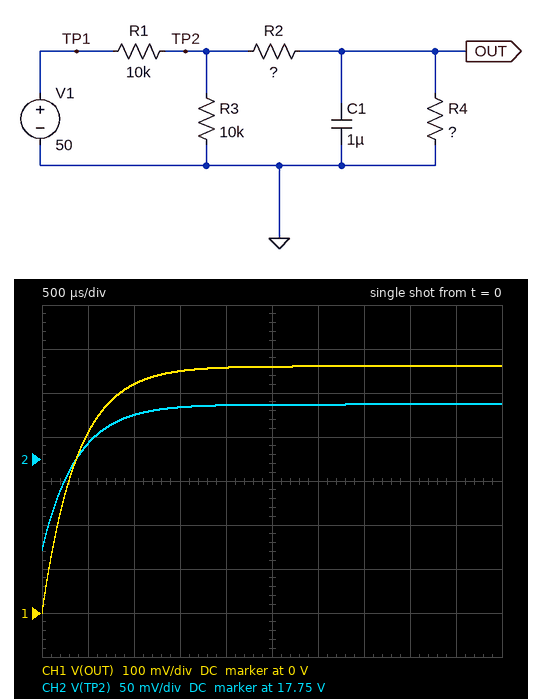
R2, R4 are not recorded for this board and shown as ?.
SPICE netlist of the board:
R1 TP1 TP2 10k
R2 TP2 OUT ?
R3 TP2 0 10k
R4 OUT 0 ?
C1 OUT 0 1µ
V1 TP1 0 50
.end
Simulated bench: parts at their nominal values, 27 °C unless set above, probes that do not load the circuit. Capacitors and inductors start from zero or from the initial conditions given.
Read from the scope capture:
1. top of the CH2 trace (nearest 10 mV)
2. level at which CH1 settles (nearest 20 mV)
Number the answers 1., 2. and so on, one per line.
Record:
1. 17.81 V
2. 560 mV
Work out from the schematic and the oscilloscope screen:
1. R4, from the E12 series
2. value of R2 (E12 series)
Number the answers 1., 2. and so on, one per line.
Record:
1. 390 Ω
2. 12 kΩ
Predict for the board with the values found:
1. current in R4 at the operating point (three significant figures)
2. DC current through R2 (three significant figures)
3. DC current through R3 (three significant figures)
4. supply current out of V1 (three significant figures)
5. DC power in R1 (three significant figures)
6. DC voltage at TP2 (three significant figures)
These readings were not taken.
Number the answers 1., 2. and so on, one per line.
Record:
1. 1.44 mA
2. 1.44 mA
3. 1.78 mA
4. 3.22 mA
5. 104 mW
6. 17.8 V
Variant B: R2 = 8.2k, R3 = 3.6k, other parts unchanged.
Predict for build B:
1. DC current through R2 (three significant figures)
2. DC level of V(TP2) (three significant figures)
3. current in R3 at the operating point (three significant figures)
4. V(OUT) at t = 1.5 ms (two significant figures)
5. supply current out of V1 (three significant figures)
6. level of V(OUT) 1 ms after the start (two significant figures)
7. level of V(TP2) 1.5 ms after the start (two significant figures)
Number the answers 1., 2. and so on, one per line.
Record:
1. 1.18 mA
2. 10.1 V
3. 2.81 mA
4. 450 mV
5. 3.99 mA
6. 430 mV
7. 10 V
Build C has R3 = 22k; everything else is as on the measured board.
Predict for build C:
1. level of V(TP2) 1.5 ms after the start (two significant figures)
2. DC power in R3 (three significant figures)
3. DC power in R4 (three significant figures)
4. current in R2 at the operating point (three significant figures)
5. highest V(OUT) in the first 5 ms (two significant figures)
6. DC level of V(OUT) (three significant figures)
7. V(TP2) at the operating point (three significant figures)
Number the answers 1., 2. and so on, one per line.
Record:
1. 22 V
2. 22.2 mW
3. 1.24 mW
4. 1.78 mA
5. 700 mV
6. 696 mV
7. 22.1 V
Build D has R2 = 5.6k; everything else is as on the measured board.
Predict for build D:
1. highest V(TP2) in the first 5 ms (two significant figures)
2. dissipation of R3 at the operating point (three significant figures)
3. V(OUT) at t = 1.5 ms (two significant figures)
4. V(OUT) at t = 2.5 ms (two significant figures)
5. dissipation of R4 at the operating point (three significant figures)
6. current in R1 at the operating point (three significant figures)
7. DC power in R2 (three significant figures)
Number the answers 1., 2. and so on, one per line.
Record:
1. 14 V
2. 18.6 mW
3. 870 mV
4. 890 mV
5. 2.02 mW
6. 3.64 mA
7. 29.0 mW
